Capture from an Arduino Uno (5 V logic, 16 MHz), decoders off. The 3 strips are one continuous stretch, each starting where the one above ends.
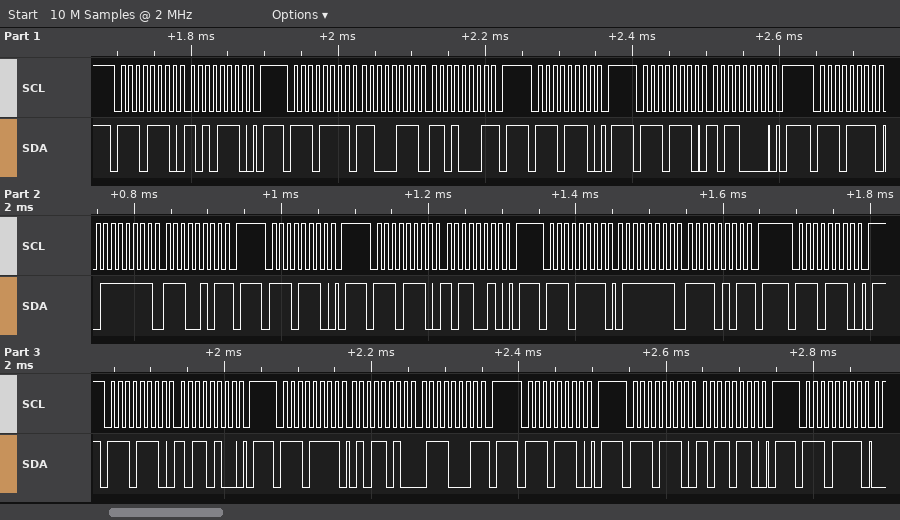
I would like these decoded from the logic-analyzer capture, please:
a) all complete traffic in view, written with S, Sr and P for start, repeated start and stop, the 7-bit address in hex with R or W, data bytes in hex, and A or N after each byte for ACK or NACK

S 77W A AE A P S 77R A C7 A D1 N P S 77W A P S 77W A B0 A P S 77R A 7F A E5 N P S 77W A P S 77W A B2 A P S 77R A 7F A F5 N P S 77W A P S 77W A B4 A P S 77R A 5A A 71 N P S 77W A P S 77W A B6 A P S 77R A
